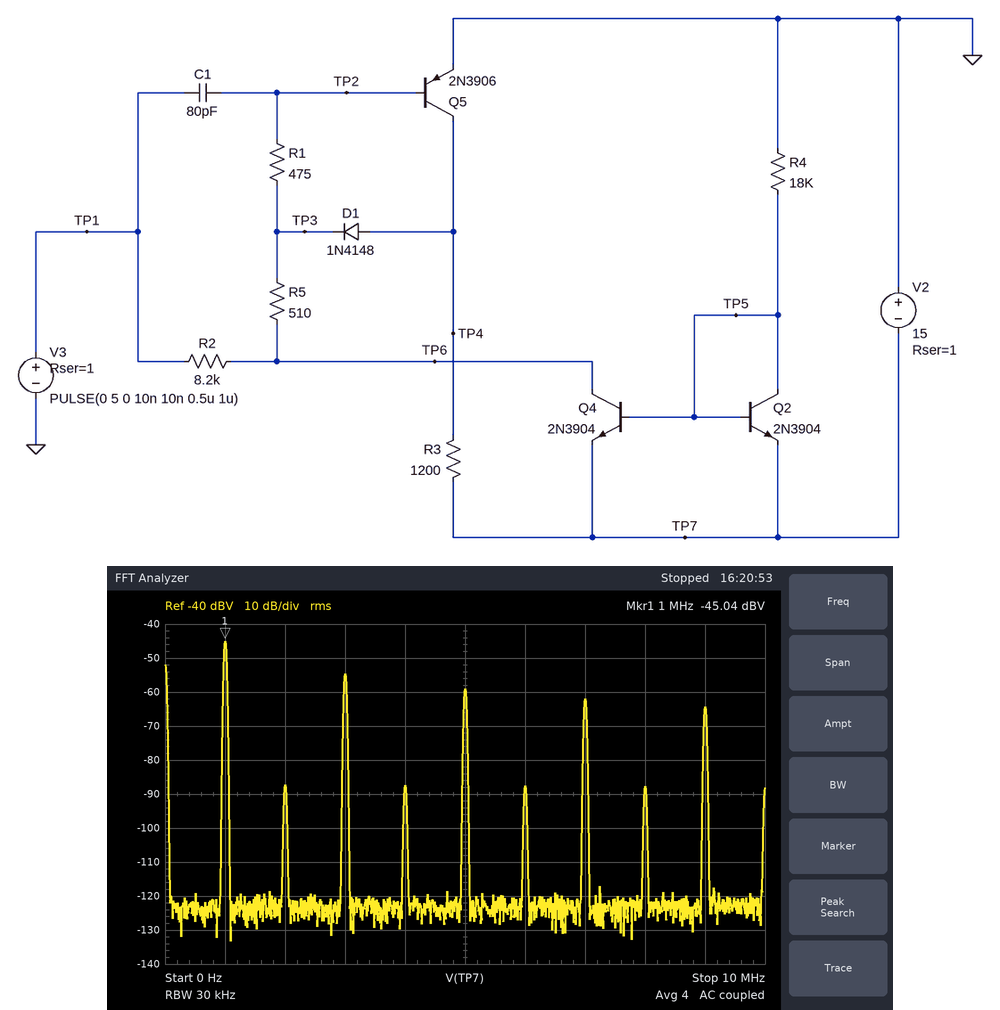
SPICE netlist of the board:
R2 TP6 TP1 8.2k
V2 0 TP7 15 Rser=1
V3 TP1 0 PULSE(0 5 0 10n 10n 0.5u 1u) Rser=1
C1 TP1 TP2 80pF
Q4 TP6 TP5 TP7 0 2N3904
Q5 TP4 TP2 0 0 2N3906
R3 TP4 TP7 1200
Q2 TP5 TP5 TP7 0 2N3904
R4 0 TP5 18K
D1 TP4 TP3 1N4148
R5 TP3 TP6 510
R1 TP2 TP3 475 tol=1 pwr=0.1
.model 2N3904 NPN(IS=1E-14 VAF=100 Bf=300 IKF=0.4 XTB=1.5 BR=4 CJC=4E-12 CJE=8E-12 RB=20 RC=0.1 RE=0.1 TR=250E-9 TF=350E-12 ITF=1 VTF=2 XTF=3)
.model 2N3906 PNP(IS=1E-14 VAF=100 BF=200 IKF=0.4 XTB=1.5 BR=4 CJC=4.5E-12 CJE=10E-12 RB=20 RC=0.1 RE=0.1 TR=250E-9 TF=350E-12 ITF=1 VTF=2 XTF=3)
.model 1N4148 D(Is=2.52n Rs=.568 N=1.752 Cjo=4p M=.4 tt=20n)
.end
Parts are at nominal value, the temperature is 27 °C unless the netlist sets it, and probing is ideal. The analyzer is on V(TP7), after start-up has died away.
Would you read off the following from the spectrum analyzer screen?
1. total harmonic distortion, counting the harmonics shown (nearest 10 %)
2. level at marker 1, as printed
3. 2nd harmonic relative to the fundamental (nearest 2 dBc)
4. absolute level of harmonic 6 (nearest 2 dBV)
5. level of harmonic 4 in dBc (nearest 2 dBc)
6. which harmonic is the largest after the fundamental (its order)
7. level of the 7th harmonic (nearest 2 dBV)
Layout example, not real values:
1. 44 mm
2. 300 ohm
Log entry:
1. 40 %
2. -45.04 dBV
3. -42 dBc
4. -88 dBV
5. -42 dBc
6. 3
7. -62 dBV
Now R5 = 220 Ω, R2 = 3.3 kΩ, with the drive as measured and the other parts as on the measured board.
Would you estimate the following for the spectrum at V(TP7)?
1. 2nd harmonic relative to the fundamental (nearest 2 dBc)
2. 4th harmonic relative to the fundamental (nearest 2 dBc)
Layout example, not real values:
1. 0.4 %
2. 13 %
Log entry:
1. -30 dBc
2. -30 dBc
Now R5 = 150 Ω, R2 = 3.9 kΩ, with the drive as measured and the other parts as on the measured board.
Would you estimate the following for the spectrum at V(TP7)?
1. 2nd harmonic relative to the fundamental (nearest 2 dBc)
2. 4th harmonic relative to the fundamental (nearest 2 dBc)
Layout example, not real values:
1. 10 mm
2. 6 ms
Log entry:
1. -32 dBc
2. -32 dBc
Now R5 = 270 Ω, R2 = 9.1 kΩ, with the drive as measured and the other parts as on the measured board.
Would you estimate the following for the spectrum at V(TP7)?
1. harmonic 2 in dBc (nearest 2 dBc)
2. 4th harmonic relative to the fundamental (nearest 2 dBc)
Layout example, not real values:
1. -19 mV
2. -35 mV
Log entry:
1. -36 dBc
2. -36 dBc
